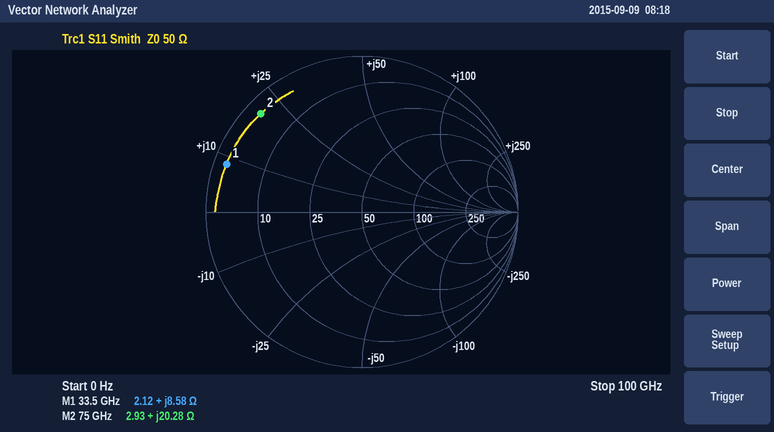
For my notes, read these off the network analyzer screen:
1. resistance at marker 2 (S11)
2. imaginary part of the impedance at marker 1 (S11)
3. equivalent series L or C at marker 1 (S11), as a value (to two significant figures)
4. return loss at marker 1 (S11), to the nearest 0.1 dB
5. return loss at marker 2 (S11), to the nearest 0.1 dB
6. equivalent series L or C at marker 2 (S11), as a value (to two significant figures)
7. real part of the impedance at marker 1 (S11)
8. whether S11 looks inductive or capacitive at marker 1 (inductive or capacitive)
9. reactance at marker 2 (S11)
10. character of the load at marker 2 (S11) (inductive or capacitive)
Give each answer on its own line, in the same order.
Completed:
2.93 Ω
+8.58 Ω
41 pH
0.7 dB
0.9 dB
43 pH
2.12 Ω
inductive
+20.28 Ω
inductive
